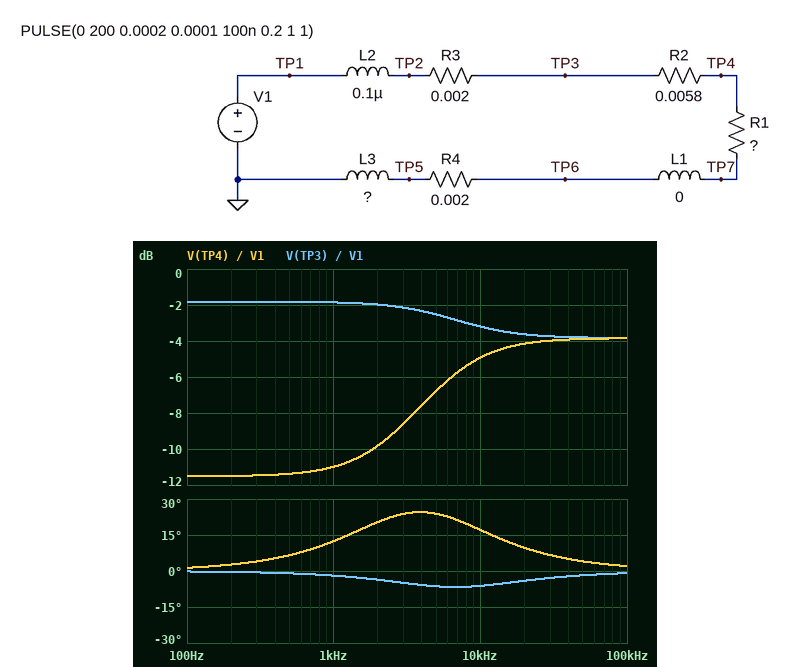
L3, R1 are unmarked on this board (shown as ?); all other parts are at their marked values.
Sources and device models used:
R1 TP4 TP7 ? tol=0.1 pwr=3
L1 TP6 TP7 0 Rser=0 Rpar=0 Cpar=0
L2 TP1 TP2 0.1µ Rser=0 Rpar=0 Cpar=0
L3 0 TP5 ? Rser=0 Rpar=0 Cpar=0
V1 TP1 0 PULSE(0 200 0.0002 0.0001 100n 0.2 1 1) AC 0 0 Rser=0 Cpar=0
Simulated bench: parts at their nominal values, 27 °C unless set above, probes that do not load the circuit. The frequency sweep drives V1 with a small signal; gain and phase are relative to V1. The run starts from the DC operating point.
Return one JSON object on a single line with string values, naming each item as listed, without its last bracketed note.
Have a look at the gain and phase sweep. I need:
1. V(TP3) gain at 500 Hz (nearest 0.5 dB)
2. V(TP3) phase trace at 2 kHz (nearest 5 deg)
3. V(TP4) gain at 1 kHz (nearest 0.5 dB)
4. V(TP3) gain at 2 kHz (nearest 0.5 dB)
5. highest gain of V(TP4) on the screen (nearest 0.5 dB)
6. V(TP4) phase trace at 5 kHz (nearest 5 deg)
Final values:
{"V(TP3) gain at 500 Hz": "-2.0 dB", "V(TP3) phase trace at 2 kHz": "-5 deg", "V(TP4) gain at 1 kHz": "-11.0 dB", "V(TP3) gain at 2 kHz": "-2.0 dB", "highest gain of V(TP4) on the screen": "-4.0 dB", "V(TP4) phase trace at 5 kHz": "25 deg"}
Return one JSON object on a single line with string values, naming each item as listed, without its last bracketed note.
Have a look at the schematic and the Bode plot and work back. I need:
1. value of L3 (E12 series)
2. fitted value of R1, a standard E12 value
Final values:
{"value of L3": "180 nH", "fitted value of R1, a standard E12 value": "820 µΩ"}
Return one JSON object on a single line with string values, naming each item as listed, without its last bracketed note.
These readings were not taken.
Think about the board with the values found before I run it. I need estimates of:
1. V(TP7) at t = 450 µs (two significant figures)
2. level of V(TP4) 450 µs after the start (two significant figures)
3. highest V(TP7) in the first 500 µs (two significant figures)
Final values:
{"V(TP7) at t = 450 µs": "38 V", "level of V(TP4) 450 µs after the start": "53 V", "highest V(TP7) in the first 500 µs": "61 V"}
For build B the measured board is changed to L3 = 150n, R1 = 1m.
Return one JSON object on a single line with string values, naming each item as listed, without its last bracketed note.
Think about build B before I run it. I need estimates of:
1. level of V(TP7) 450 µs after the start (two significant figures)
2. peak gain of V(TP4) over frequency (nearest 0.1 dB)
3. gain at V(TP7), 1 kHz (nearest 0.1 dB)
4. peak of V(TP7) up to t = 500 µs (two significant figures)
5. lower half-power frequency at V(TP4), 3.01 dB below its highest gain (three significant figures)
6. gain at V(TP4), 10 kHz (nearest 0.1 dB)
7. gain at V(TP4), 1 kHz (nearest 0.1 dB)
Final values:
{"level of V(TP7) 450 µs after the start": "37 V", "peak gain of V(TP4) over frequency": "-4.4 dB", "gain at V(TP7), 1 kHz": "-13.9 dB", "peak of V(TP7) up to t = 500 µs": "56 V", "lower half-power frequency at V(TP4), 3.01 dB below its highest gain": "5.20 kHz", "gain at V(TP4), 10 kHz": "-5.7 dB", "gain at V(TP4), 1 kHz": "-10.8 dB"}
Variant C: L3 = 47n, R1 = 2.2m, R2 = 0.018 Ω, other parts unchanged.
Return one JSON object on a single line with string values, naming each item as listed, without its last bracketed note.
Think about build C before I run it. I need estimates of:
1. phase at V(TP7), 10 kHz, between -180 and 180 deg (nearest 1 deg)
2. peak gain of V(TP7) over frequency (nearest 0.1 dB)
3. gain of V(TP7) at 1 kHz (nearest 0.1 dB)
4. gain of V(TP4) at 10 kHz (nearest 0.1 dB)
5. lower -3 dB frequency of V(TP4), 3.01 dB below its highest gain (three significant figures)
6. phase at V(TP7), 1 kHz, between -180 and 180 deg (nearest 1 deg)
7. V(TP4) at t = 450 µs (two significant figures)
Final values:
{"phase at V(TP7), 10 kHz, between -180 and 180 deg": "35 deg", "peak gain of V(TP7) over frequency": "-9.9 dB", "gain of V(TP7) at 1 kHz": "-21.6 dB", "gain of V(TP4) at 10 kHz": "-14.1 dB", "lower -3 dB frequency of V(TP4), 3.01 dB below its highest gain": "16.8 kHz", "phase at V(TP7), 1 kHz, between -180 and 180 deg": "6 deg", "V(TP4) at t = 450 µs": "35 V"}
